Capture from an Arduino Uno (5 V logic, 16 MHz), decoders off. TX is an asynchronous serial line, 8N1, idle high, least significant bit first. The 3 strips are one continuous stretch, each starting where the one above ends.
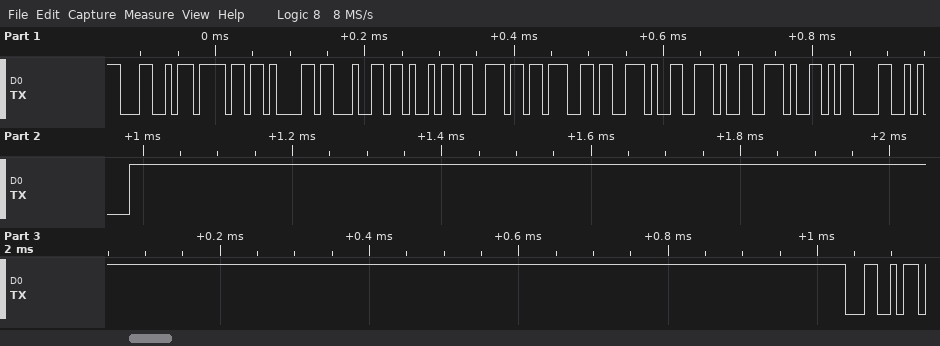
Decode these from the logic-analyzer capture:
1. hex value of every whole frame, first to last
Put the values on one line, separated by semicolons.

0x4C 0x6F 0x61 0x64 0x69 0x6E 0x67 0x2E 0x2E 0x2E 0x0D 0x0A 0x4C
